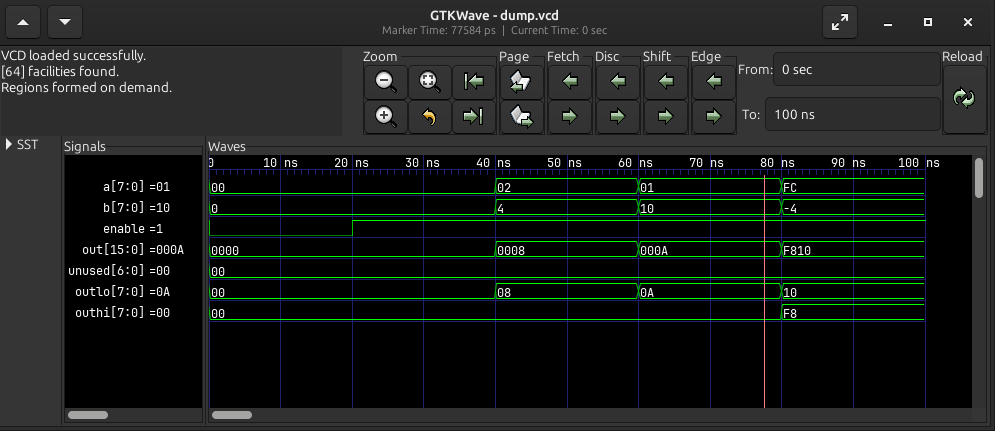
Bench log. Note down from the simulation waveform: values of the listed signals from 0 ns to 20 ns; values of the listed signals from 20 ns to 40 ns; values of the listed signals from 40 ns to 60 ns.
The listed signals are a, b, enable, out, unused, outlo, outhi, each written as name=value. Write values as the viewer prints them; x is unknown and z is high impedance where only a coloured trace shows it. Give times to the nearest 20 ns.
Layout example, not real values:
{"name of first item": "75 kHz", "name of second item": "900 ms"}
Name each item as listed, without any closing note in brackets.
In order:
{"values of the listed signals from 0 ns to 20 ns": "a=00, b=0, enable=0, out=0000, unused=00, outlo=00, outhi=00", "values of the listed signals from 20 ns to 40 ns": "a=00, b=0, enable=1, out=0000, unused=00, outlo=00, outhi=00", "values of the listed signals from 40 ns to 60 ns": "a=02, b=4, enable=1, out=0008, unused=00, outlo=08, outhi=00"}
